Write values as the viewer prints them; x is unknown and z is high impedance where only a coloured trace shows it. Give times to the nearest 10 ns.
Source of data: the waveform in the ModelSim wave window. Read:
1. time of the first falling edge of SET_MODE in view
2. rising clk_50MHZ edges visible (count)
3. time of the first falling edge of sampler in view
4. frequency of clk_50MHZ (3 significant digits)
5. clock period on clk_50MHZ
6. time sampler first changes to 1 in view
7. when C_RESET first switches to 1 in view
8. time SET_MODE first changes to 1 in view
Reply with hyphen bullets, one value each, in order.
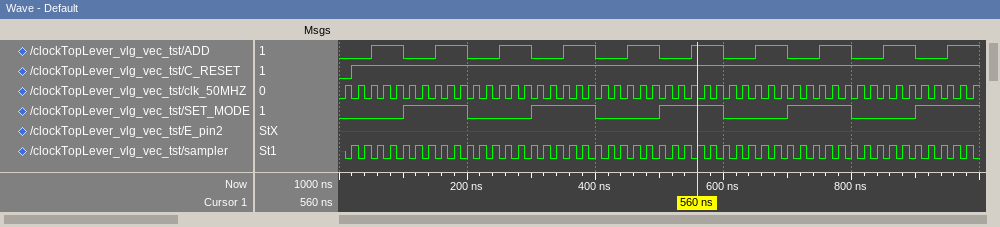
- 200 ns
- 50
- 30 ns
- 50.0 MHz
- 20 ns
- 20 ns
- 20 ns
- 100 ns
